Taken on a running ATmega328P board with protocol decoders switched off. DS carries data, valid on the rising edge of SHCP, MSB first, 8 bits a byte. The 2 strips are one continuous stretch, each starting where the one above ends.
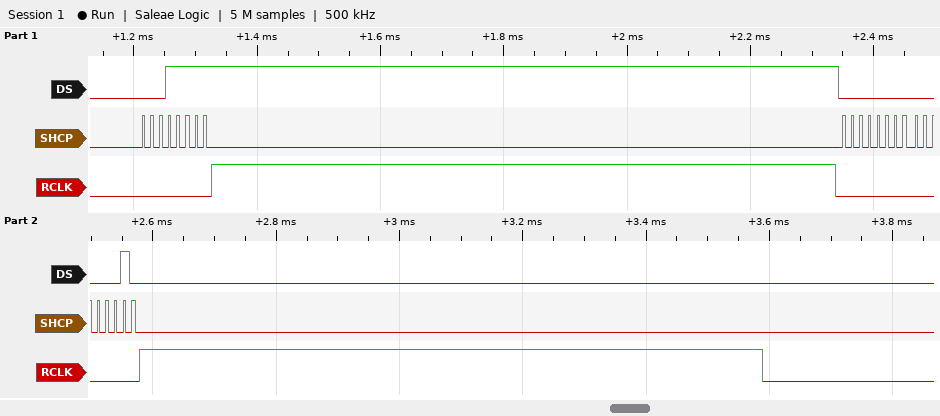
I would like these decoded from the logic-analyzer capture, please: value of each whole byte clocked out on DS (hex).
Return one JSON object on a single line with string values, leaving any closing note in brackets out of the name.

{"value of each whole byte clocked out on DS": "1F 00 02"}
